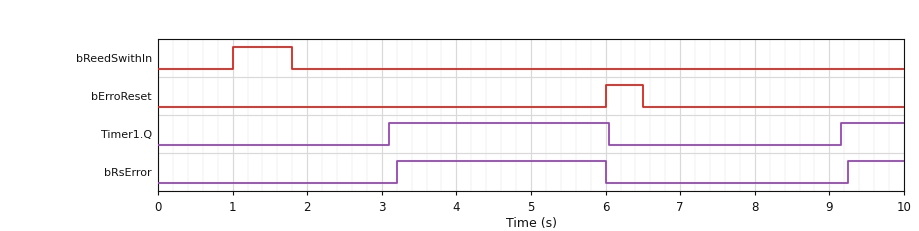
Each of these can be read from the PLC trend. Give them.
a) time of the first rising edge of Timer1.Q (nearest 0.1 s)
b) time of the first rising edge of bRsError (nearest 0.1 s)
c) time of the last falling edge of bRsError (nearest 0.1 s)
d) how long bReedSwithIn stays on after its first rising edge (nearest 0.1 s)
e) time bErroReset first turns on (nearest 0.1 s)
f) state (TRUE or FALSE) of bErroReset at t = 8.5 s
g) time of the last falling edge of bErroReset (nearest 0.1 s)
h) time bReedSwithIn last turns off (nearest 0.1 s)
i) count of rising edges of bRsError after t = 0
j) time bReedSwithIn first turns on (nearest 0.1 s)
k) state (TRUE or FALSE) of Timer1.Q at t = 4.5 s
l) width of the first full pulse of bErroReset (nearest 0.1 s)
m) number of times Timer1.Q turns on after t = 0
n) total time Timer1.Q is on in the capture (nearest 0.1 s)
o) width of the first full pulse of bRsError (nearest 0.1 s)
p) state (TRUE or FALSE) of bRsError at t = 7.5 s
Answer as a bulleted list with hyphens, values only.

- 3.1 s
- 3.2 s
- 6.0 s
- 0.8 s
- 6.0 s
- FALSE
- 6.5 s
- 1.8 s
- 2
- 1.0 s
- TRUE
- 0.5 s
- 2
- 3.8 s
- 2.8 s
- FALSE
